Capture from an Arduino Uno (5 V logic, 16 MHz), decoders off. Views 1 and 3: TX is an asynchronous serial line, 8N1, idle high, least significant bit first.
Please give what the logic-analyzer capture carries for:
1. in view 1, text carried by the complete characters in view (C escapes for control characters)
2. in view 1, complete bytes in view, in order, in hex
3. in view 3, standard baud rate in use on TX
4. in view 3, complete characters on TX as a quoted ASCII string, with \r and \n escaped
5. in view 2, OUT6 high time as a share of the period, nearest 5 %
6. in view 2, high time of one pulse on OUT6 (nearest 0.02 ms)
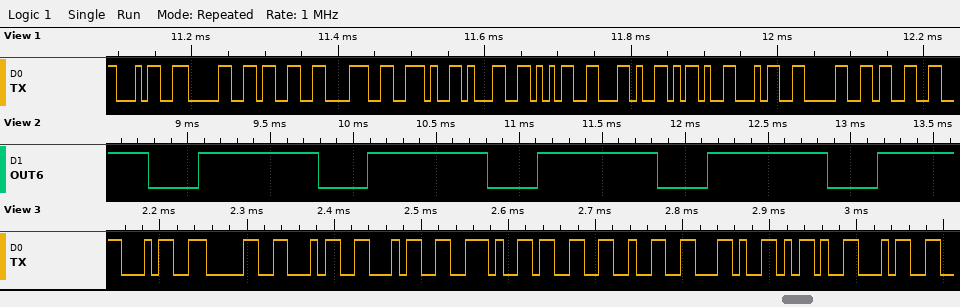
"4038.15,-403"
0x34 0x30 0x33 0x38 0x2E 0x31 0x35 0x2C 0x2D 0x34 0x30 0x33
115200 baud
"4044.32,-4"
70 %
0.72 ms
